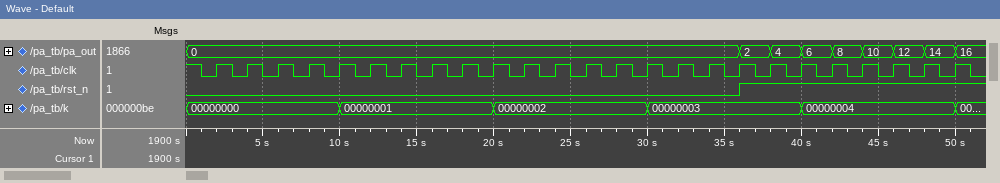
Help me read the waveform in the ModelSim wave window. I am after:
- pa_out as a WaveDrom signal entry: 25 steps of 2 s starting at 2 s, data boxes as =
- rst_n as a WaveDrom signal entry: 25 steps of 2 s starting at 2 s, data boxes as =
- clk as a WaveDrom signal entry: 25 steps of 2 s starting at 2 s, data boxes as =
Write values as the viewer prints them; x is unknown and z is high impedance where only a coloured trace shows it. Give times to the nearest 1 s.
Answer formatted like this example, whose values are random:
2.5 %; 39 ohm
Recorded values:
{name: 'pa_out', wave: '=................========', data: '0 2 4 6 8 10 12 14 16'}; {name: 'rst_n', wave: '0................1.......'}; {name: 'clk', wave: 'p........................'}
